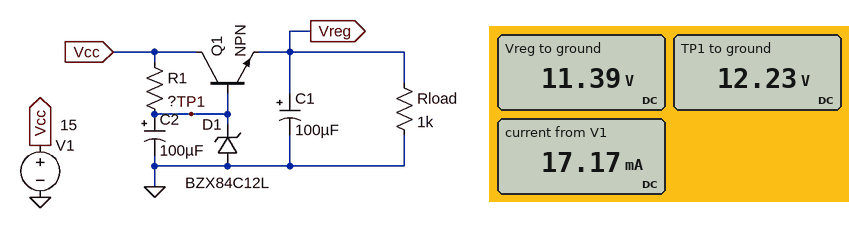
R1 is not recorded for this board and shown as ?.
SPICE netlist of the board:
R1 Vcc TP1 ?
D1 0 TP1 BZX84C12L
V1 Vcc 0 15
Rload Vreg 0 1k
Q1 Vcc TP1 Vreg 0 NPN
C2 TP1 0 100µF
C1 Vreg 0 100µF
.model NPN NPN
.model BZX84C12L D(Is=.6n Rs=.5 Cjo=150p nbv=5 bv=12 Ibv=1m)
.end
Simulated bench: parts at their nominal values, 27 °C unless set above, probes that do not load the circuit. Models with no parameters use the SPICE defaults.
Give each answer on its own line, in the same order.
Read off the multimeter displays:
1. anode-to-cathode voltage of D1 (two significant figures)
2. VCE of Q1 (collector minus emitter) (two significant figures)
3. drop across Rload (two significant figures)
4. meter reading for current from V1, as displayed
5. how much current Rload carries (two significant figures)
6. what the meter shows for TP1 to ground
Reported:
-12 V
3.6 V
11 V
17.17 mA
11 mA
12.23 V
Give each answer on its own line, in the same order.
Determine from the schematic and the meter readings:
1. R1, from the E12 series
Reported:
470 Ω
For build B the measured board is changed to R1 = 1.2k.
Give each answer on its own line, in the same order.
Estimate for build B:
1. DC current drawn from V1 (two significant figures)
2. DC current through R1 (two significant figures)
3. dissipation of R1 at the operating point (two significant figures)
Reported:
14 mA
2.4 mA
7.0 mW
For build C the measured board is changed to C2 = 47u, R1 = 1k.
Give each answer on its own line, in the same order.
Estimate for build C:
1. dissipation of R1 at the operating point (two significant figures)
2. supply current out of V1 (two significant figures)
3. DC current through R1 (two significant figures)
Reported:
8.2 mW
14 mA
2.9 mA
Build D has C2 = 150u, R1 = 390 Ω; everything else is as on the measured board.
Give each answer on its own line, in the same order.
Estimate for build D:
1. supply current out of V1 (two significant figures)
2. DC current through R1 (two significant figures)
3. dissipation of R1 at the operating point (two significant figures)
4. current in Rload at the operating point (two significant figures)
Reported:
18 mA
7.0 mA
19 mW
11 mA
